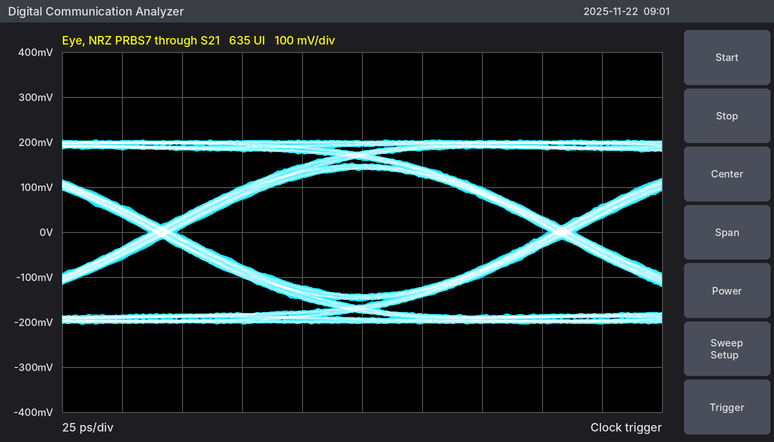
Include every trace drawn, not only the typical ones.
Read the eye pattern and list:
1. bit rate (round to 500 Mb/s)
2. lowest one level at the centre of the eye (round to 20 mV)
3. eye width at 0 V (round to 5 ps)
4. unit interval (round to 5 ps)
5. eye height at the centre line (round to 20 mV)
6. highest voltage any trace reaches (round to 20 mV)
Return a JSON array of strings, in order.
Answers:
["6.0 Gb/s", "140 mV", "155 ps", "165 ps", "280 mV", "200 mV"]
